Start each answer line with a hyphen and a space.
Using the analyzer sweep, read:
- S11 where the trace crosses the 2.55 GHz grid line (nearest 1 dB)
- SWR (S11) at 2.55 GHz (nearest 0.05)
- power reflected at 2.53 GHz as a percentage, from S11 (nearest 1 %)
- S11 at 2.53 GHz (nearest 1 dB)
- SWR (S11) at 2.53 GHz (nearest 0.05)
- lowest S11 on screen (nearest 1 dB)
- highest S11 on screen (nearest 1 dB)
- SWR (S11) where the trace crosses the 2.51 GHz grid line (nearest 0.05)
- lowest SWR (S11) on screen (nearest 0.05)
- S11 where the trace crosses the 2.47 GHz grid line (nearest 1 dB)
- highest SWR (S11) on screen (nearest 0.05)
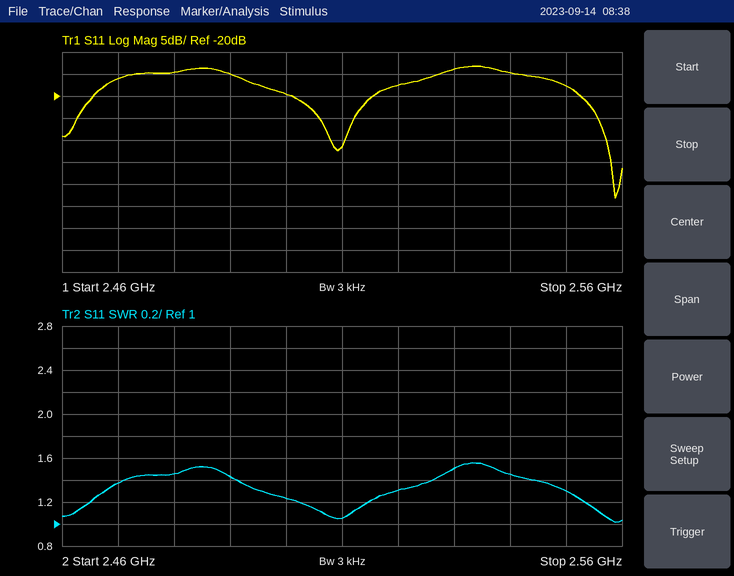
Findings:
- -18 dB
- 1.30
- 4 %
- -14 dB
- 1.50
- -43 dB
- -13 dB
- 1.05
- 1.00
- -16 dB
- 1.55
